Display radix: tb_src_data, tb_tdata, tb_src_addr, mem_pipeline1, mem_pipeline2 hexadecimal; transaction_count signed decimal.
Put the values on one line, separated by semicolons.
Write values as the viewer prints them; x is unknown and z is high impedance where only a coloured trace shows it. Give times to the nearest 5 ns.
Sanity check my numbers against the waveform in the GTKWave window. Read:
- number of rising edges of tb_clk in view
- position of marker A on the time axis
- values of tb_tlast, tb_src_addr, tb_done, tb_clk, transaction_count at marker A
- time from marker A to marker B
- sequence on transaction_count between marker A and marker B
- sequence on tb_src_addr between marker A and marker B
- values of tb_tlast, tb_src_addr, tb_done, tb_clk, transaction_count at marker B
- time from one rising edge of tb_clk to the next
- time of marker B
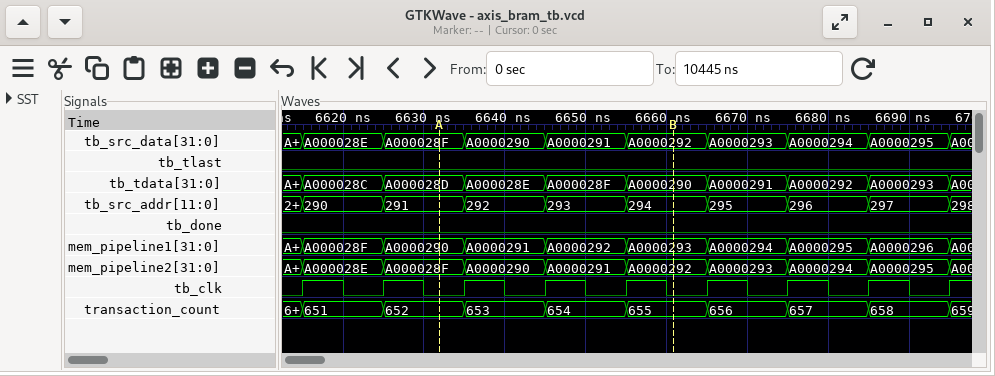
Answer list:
9; 6630 ns; tb_tlast=0, tb_src_addr=291, tb_done=0, tb_clk=0, transaction_count=652; 30 ns; 652, 653, 654, 655; 291, 292, 293, 294; tb_tlast=0, tb_src_addr=294, tb_done=0, tb_clk=0, transaction_count=655; 10 ns; 6660 ns
